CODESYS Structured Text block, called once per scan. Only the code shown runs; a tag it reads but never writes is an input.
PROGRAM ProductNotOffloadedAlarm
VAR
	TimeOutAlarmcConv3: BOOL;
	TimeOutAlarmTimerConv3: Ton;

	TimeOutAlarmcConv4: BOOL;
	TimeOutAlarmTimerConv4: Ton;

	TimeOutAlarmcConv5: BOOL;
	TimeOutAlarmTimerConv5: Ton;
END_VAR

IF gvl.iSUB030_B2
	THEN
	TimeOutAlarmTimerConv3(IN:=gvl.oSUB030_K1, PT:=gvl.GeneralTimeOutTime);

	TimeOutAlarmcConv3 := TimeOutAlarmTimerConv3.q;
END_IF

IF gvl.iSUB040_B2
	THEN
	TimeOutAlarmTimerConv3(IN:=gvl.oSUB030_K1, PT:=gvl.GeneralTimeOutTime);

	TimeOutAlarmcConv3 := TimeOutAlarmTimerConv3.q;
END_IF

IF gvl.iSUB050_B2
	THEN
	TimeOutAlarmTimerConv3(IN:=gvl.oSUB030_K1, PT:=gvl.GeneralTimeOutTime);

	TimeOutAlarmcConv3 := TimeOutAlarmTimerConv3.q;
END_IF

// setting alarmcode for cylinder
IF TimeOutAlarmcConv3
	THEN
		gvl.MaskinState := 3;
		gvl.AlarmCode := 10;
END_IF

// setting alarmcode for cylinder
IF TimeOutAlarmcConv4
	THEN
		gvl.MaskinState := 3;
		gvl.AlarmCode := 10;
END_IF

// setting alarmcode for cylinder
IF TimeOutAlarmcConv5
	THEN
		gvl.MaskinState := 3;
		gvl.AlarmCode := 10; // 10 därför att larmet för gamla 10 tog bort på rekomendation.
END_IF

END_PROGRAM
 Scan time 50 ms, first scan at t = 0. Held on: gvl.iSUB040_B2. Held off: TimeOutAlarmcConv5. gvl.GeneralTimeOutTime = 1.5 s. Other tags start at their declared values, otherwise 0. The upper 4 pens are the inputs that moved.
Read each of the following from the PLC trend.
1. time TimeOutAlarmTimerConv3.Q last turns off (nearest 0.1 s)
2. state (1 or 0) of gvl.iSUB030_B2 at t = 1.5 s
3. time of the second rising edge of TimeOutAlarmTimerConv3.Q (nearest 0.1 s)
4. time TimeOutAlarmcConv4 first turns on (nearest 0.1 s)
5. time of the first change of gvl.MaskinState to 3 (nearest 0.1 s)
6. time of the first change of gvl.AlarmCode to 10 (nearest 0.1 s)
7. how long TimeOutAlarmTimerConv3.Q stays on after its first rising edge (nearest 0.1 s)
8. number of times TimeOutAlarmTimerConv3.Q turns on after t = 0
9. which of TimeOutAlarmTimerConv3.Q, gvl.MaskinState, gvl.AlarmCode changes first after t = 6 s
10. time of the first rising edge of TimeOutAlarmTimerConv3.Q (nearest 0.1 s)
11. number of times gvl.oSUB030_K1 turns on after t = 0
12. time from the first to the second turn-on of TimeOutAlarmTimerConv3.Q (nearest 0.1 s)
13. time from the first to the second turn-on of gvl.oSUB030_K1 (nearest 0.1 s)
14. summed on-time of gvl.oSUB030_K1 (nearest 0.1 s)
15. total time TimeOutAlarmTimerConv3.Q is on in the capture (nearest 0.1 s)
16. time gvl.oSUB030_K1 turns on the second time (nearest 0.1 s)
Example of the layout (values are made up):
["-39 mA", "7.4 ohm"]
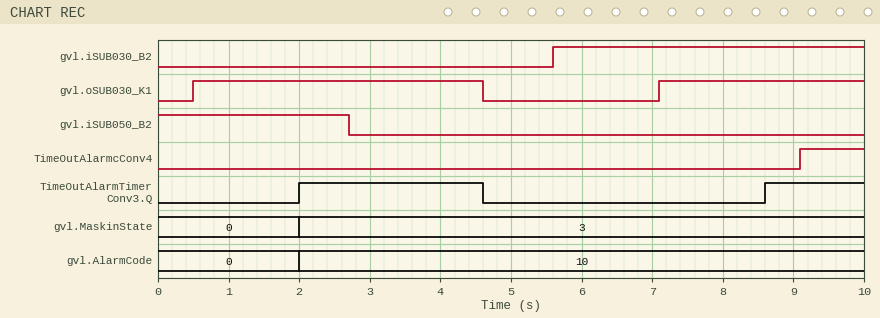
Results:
["4.6 s", "0", "8.6 s", "9.1 s", "2.0 s", "2.0 s", "2.6 s", "2", "TimeOutAlarmTimerConv3.Q", "2.0 s", "2", "6.6 s", "6.6 s", "7.0 s", "4.0 s", "7.1 s"]
